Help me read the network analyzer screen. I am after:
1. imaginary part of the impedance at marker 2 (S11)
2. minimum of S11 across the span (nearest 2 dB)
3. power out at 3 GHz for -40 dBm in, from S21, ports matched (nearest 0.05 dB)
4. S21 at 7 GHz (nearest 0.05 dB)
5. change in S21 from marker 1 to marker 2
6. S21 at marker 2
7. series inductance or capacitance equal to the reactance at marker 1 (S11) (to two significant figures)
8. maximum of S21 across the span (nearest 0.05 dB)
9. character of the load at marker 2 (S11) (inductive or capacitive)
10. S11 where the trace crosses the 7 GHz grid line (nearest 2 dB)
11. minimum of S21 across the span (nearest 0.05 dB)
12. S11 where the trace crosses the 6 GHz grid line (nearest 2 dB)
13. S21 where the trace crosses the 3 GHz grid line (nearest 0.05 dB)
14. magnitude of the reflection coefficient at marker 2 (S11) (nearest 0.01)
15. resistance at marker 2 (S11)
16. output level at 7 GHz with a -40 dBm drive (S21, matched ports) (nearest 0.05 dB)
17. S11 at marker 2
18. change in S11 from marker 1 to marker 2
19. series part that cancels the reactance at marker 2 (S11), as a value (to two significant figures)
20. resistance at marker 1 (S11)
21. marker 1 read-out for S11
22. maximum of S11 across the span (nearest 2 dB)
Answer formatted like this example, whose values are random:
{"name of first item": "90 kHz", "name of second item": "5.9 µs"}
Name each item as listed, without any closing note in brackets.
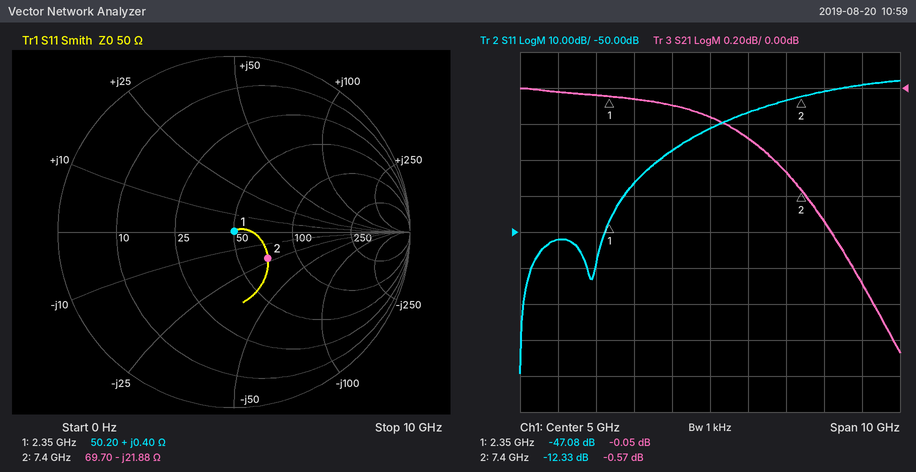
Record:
{"imaginary part of the impedance at marker 2": "-21.88 Ω", "minimum of S11 across the span": "-90 dB", "power out at 3 GHz for -40 dBm in, from S21, ports matched": "-40.05 dBm", "S21 at 7 GHz": "-0.45 dB", "change in S21 from marker 1 to marker 2": "-0.52 dB", "S21 at marker 2": "-0.57 dB", "series inductance or capacitance equal to the reactance at marker 1 (S11)": "27 pH", "maximum of S21 across the span": "0.00 dB", "character of the load at marker 2 (S11)": "capacitive", "S11 where the trace crosses the 7 GHz grid line": "-14 dB", "minimum of S21 across the span": "-1.45 dB", "S11 where the trace crosses the 6 GHz grid line": "-16 dB", "S21 where the trace crosses the 3 GHz grid line": "-0.05 dB", "magnitude of the reflection coefficient at marker 2 (S11)": "0.24", "resistance at marker 2": "69.70 Ω", "output level at 7 GHz with a -40 dBm drive (S21, matched ports)": "-40.45 dBm", "S11 at marker 2": "-12.33 dB", "change in S11 from marker 1 to marker 2": "34.75 dB", "series part that cancels the reactance at marker 2 (S11), as a value": "470 pH", "resistance at marker 1": "50.20 Ω", "marker 1 read-out for S11": "-47.08 dB", "maximum of S11 across the span": "-8 dB"}
